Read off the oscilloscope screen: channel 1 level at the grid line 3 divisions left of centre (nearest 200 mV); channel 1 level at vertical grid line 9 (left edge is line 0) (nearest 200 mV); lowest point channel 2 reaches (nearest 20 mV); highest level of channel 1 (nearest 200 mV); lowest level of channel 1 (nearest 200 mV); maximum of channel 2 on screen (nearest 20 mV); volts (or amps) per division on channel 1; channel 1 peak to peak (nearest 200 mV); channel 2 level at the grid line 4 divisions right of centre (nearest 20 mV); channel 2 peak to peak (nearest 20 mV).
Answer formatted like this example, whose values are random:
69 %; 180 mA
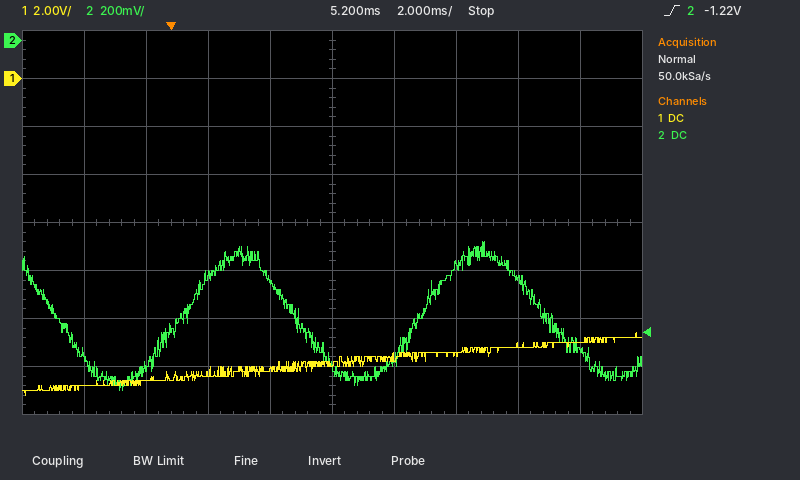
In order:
-12.6 V; -11.0 V; -1.46 V; -10.6 V; -13.2 V; -840 mV; 2 V; 2.6 V; -1.30 V; 620 mV
